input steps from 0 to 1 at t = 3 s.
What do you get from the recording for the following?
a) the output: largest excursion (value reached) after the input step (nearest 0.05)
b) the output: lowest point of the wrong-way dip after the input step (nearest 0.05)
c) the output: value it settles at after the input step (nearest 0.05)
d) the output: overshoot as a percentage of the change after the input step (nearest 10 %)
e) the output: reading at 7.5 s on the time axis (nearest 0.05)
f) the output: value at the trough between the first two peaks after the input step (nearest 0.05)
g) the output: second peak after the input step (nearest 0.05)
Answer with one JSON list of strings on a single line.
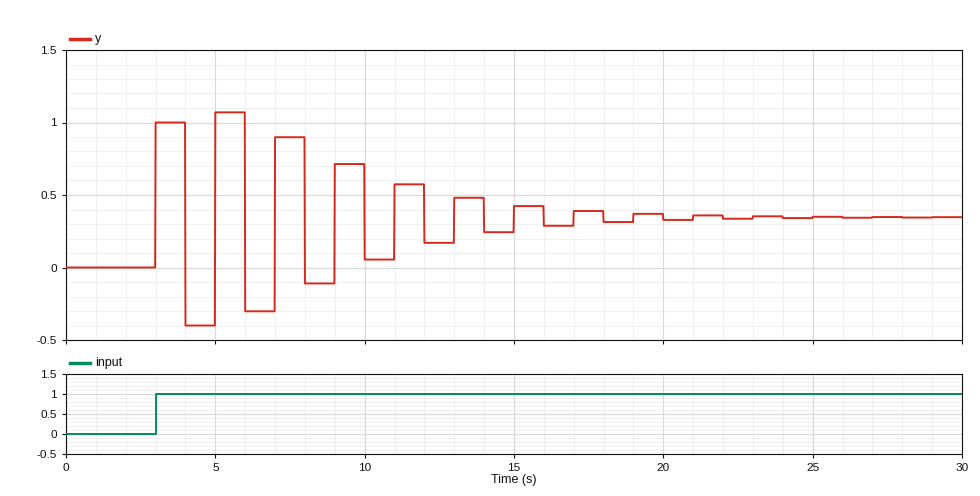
["1.05", "-0.40", "0.35", "210 %", "0.90", "-0.30", "0.90"]
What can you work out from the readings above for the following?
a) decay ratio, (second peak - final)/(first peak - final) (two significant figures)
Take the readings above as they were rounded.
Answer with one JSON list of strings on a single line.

["0.79"]
